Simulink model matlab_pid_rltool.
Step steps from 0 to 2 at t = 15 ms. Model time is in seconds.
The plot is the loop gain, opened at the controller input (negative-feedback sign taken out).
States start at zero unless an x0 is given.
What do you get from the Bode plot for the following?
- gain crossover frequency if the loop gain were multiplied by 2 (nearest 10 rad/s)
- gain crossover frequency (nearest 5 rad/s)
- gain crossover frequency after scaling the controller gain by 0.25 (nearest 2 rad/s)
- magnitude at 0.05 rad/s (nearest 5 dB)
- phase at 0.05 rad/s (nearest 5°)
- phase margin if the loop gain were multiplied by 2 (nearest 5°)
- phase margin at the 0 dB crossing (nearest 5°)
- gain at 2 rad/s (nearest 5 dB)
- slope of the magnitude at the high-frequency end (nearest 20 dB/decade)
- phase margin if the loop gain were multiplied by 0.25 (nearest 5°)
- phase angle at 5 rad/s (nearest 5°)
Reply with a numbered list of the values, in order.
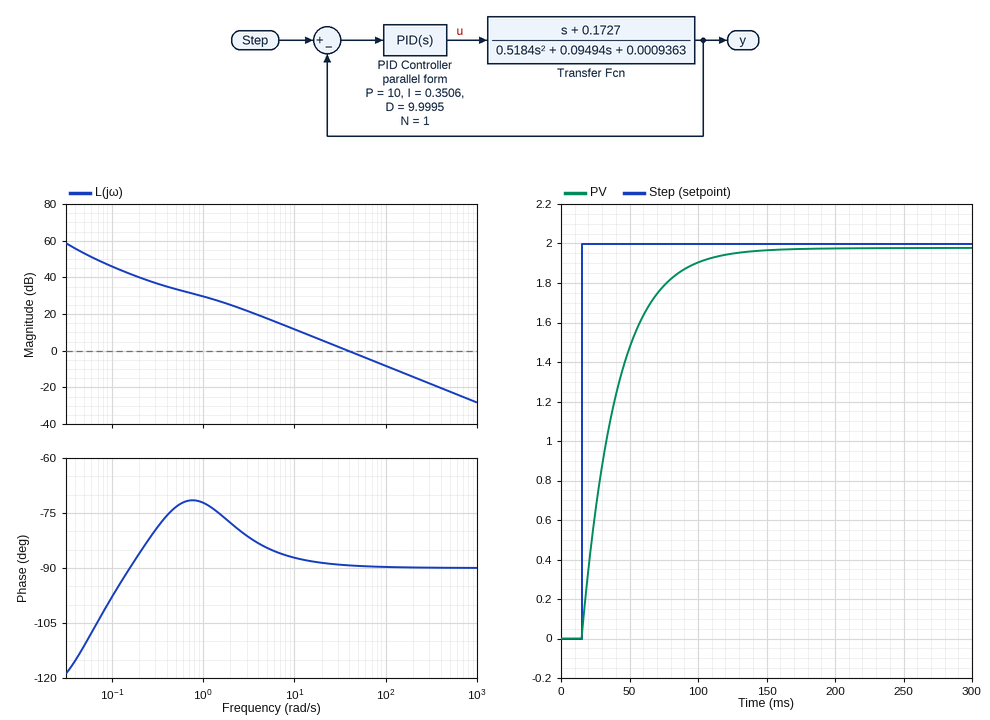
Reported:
1. 80 rad/s
2. 40 rad/s
3. 10 rad/s
4. 55 dB
5. -110°
6. 90°
7. 90°
8. 25 dB
9. -20 dB/decade
10. 95°
11. -85°
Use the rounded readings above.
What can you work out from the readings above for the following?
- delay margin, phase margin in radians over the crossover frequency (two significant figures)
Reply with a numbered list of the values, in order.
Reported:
1. 0.039 s
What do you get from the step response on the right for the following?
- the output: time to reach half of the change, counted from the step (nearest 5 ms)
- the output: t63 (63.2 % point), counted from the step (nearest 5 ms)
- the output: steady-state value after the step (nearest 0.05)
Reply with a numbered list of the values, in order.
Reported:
1. 20 ms
2. 25 ms
3. 2.00
